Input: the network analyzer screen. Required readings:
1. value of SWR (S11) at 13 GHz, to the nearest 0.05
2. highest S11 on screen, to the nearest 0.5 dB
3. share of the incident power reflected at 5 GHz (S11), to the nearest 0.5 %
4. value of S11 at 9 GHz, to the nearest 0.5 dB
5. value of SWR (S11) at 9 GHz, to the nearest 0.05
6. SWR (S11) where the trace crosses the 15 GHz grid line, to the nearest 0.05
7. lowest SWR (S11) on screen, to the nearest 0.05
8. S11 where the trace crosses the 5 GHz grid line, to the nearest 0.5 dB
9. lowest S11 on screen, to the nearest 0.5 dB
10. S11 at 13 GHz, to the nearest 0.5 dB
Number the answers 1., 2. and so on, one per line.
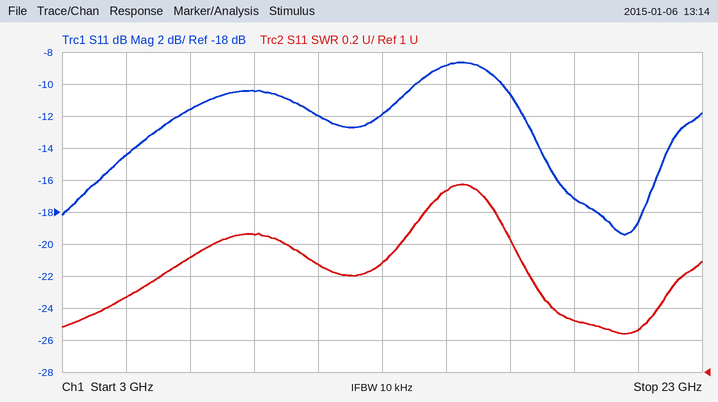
1. 1.70
2. -8.5 dB
3. 3.5 %
4. -10.5 dB
5. 1.85
6. 2.15
7. 1.25
8. -14.5 dB
9. -19.5 dB
10. -12.0 dB
